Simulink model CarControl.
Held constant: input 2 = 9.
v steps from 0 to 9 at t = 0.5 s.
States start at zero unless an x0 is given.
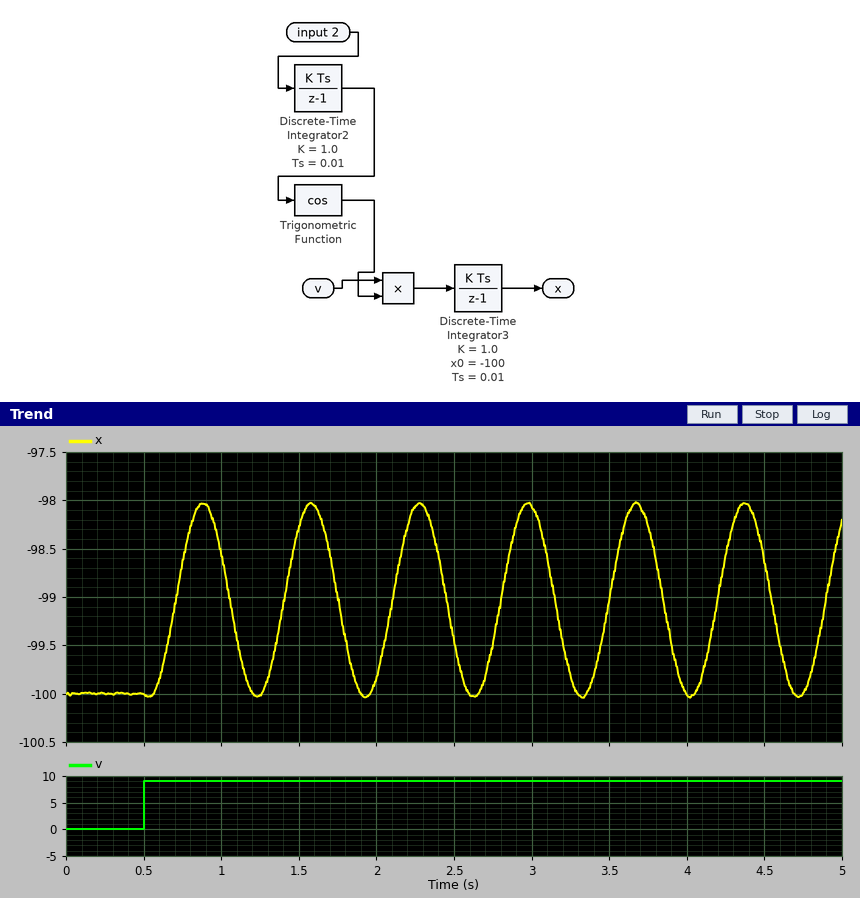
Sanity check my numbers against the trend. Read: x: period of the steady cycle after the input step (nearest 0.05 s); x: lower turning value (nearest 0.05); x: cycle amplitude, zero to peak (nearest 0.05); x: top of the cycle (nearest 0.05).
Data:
0.70 s
-100.05
1.00
-98.05
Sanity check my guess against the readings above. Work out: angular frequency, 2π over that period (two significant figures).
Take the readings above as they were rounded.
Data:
9.0 rad/s
